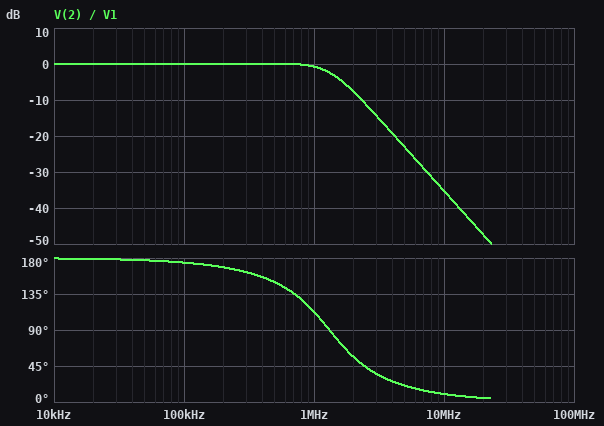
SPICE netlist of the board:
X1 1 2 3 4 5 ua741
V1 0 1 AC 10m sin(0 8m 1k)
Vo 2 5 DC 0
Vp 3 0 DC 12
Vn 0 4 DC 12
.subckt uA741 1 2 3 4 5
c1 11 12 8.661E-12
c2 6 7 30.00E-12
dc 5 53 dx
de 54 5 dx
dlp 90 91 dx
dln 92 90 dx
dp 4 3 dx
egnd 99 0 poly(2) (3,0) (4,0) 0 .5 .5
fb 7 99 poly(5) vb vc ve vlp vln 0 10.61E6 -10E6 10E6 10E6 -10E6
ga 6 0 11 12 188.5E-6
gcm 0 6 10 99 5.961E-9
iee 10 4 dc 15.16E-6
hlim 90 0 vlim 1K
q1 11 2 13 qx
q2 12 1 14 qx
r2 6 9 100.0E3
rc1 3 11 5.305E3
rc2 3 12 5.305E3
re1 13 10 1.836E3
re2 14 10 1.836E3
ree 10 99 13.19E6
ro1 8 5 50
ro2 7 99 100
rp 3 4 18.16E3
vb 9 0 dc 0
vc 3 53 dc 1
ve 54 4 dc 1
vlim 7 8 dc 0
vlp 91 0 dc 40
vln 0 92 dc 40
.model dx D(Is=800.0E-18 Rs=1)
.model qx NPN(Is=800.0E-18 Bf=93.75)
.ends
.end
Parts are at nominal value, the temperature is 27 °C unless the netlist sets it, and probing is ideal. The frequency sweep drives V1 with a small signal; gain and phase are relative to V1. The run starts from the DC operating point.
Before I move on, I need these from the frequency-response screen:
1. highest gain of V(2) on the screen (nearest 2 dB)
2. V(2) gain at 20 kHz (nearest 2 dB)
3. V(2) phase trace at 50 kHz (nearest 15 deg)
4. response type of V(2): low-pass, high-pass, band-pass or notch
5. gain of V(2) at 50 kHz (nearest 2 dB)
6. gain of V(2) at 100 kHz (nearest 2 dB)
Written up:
0 dB
0 dB
180 deg
low-pass
0 dB
0 dB
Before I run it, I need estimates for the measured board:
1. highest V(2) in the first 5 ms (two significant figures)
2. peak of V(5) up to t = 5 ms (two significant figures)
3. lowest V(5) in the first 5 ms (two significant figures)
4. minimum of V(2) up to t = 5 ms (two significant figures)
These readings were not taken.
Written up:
8.0 mV
8.0 mV
-8.0 mV
-8.0 mV
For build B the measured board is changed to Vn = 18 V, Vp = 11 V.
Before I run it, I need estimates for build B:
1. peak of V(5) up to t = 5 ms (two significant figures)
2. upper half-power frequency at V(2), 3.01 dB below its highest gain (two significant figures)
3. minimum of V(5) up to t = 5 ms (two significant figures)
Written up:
7.9 mV
1.4 MHz
-8.1 mV
